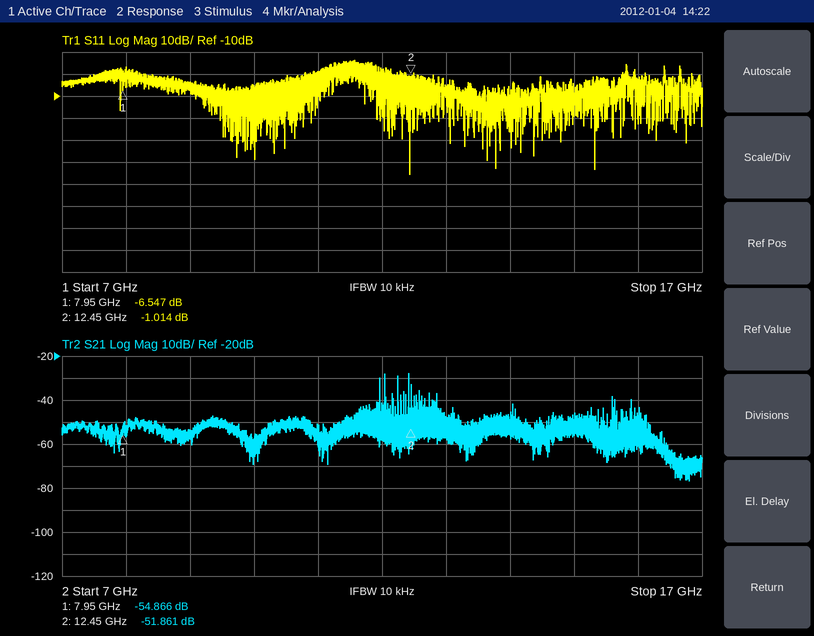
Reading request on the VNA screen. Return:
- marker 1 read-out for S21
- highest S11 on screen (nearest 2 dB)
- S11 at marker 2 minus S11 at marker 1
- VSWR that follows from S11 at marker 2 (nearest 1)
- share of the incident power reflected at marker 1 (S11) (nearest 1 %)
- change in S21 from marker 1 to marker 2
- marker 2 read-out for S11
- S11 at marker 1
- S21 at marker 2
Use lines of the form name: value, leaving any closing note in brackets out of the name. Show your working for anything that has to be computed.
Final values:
marker 1 read-out for S21: -54.866 dB
highest S11 on screen: 6 dB
S11 at marker 2 minus S11 at marker 1: -1.014 − (-6.547) = 5.533 dB
VSWR that follows from S11 at marker 2: (1 + 0.8898)/(1 − 0.8898) ≈ 17
share of the incident power reflected at marker 1 (S11): 10^(-6.547/10) ≈ 22 %
change in S21 from marker 1 to marker 2: -51.861 − (-54.866) = 3.005 dB
marker 2 read-out for S11: -1.014 dB
S11 at marker 1: -6.547 dB
S21 at marker 2: -51.861 dB
